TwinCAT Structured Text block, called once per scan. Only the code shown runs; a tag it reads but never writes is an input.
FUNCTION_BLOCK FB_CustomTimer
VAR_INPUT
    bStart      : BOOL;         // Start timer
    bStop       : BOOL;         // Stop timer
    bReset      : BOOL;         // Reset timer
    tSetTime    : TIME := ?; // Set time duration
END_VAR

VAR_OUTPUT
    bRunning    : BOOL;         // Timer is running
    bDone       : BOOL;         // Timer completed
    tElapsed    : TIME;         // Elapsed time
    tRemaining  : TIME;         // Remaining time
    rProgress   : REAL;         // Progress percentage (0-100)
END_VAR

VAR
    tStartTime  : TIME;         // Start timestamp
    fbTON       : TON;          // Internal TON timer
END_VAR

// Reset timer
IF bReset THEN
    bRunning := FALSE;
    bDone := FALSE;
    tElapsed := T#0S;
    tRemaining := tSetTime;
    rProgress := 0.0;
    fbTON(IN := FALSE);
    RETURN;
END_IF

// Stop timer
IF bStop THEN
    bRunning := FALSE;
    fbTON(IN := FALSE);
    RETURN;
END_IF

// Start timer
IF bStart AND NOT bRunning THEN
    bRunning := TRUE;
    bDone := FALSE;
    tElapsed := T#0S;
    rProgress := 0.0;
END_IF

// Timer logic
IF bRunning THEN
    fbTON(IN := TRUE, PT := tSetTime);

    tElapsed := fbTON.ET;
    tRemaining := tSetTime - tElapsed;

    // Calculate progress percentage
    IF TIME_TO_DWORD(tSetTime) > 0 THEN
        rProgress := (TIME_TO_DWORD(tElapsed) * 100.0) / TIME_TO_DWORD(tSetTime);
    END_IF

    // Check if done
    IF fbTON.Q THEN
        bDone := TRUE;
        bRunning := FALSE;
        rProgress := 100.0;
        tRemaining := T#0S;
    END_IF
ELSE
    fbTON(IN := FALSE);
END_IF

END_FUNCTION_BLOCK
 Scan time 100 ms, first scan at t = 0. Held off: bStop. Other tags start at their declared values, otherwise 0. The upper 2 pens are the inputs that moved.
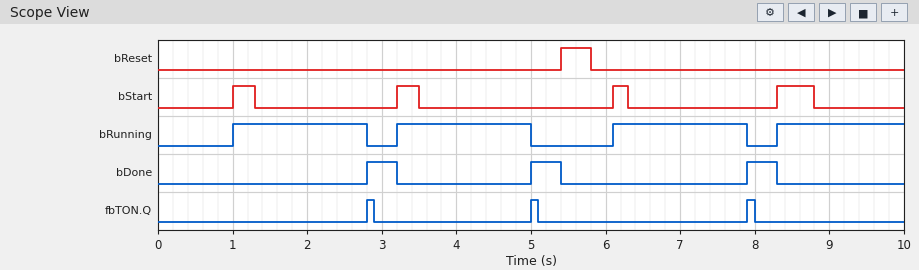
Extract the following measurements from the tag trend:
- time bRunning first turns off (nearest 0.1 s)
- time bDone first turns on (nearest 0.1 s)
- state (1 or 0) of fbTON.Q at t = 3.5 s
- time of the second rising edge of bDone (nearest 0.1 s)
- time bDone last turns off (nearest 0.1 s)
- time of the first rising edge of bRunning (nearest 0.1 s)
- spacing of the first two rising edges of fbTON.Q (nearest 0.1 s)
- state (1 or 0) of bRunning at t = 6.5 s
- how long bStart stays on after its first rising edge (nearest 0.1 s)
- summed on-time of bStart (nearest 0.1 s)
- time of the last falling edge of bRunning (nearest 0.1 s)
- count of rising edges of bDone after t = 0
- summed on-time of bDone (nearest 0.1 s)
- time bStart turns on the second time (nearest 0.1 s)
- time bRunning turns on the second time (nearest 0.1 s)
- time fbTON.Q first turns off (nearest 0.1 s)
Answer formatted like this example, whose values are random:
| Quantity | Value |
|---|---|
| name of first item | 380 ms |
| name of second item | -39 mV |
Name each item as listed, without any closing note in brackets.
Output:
| Quantity | Value |
|---|---|
| time bRunning first turns off | 2.8 s |
| time bDone first turns on | 2.8 s |
| state (1 or 0) of fbTON.Q at t = 3.5 s | 0 |
| time of the second rising edge of bDone | 5.0 s |
| time bDone last turns off | 8.3 s |
| time of the first rising edge of bRunning | 1.0 s |
| spacing of the first two rising edges of fbTON.Q | 2.2 s |
| state (1 or 0) of bRunning at t = 6.5 s | 1 |
| how long bStart stays on after its first rising edge | 0.3 s |
| summed on-time of bStart | 1.3 s |
| time of the last falling edge of bRunning | 7.9 s |
| count of rising edges of bDone after t = 0 | 3 |
| summed on-time of bDone | 1.2 s |
| time bStart turns on the second time | 3.2 s |
| time bRunning turns on the second time | 3.2 s |
| time fbTON.Q first turns off | 2.9 s |
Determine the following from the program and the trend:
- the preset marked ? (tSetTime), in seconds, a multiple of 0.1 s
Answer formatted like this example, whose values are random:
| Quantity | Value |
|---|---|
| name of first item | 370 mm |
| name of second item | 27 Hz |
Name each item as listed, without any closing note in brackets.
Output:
| Quantity | Value |
|---|---|
| the preset marked ? (tSetTime), in seconds, a multiple of 0.1 s | 1.8 s |
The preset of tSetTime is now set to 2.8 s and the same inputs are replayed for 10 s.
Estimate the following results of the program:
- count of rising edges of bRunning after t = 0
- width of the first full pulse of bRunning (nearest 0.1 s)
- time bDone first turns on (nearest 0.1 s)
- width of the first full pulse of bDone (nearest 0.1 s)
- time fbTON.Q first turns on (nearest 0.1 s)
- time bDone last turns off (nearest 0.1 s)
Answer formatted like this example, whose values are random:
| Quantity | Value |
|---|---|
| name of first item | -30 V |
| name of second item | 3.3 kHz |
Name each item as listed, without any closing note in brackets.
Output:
| Quantity | Value |
|---|---|
| count of rising edges of bRunning after t = 0 | 2 |
| width of the first full pulse of bRunning | 2.8 s |
| time bDone first turns on | 3.8 s |
| width of the first full pulse of bDone | 1.6 s |
| time fbTON.Q first turns on | 3.8 s |
| time bDone last turns off | 5.4 s |
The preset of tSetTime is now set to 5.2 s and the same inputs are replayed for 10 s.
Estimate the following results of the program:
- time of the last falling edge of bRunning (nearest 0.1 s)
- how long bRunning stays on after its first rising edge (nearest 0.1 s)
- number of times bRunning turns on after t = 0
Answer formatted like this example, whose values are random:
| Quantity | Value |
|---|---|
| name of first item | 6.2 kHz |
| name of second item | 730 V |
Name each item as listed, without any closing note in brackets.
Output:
| Quantity | Value |
|---|---|
| time of the last falling edge of bRunning | 5.4 s |
| how long bRunning stays on after its first rising edge | 4.4 s |
| number of times bRunning turns on after t = 0 | 2 |
